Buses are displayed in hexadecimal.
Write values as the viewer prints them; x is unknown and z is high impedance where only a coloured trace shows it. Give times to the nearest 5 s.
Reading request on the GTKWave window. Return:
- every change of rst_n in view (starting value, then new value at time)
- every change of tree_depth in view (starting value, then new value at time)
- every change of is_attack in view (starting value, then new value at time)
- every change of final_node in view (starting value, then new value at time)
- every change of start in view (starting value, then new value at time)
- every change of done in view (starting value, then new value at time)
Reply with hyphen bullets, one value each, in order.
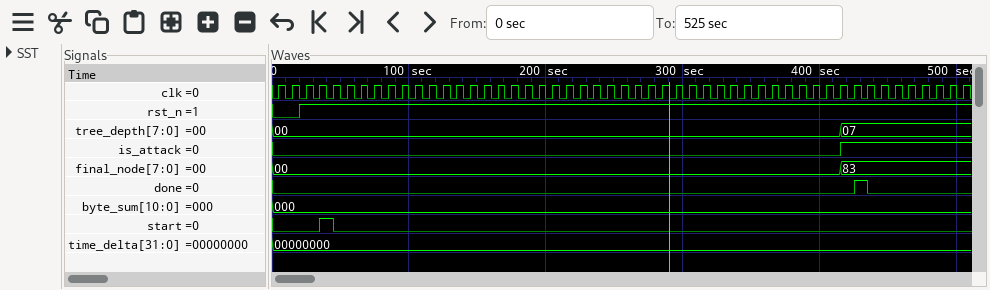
- 0, 1 at 20 s
- 00, 07 at 415 s
- 0, 1 at 415 s
- 00, 83 at 415 s
- 0, 1 at 35 s, 0 at 45 s
- 0, 1 at 425 s, 0 at 435 s
